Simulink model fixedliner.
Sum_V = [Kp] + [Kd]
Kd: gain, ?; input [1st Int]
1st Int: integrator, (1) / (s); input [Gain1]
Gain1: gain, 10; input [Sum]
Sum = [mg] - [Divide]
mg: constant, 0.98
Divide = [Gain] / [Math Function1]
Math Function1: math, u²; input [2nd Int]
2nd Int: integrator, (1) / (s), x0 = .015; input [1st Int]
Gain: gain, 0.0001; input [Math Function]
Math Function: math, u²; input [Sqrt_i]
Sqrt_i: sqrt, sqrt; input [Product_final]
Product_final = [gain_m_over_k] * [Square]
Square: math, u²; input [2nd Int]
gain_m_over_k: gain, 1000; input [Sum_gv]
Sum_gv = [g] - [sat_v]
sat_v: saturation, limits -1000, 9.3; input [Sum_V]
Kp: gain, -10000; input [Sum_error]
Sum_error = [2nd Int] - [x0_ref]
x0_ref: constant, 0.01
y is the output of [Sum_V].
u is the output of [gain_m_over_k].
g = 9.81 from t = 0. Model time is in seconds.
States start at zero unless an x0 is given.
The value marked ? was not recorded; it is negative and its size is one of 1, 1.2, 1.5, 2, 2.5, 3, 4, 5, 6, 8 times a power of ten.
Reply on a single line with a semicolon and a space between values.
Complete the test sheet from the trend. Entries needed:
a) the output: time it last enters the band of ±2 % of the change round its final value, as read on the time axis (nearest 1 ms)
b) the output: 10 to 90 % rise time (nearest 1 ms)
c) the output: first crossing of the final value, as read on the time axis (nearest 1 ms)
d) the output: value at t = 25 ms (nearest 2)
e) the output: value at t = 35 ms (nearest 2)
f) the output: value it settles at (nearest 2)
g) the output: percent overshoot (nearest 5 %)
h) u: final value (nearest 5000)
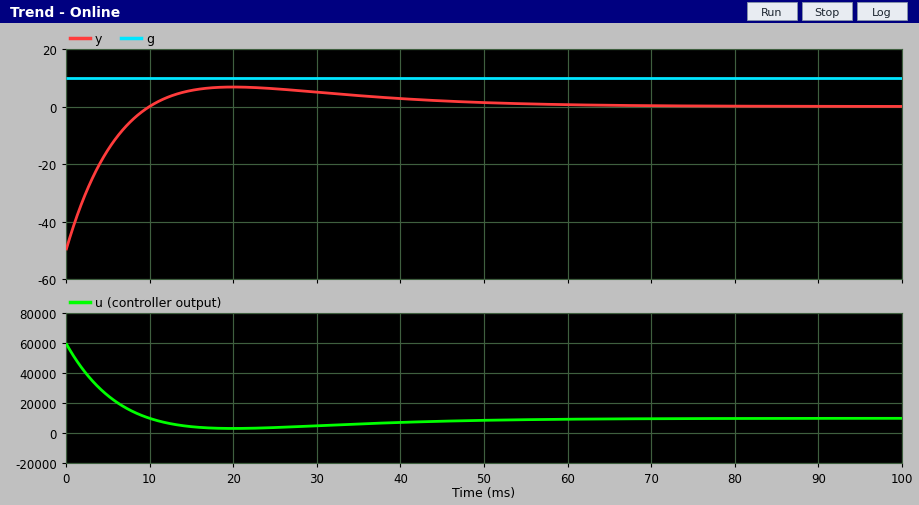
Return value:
54 ms; 7 ms; 10 ms; 6; 4; 0; 15 %; 10000
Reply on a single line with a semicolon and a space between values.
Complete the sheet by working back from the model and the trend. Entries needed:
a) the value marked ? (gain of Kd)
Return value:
-200
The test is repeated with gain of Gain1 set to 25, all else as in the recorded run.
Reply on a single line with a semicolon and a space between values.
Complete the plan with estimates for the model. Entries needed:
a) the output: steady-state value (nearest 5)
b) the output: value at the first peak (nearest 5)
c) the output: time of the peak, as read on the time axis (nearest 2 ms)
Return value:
0; 5; 10 ms
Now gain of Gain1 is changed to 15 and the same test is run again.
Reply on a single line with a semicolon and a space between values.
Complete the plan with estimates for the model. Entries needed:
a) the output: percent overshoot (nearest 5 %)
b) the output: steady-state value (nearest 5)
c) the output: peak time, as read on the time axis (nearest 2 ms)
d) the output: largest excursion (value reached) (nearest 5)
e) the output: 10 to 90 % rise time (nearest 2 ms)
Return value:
10 %; 0; 16 ms; 5; 6 ms
